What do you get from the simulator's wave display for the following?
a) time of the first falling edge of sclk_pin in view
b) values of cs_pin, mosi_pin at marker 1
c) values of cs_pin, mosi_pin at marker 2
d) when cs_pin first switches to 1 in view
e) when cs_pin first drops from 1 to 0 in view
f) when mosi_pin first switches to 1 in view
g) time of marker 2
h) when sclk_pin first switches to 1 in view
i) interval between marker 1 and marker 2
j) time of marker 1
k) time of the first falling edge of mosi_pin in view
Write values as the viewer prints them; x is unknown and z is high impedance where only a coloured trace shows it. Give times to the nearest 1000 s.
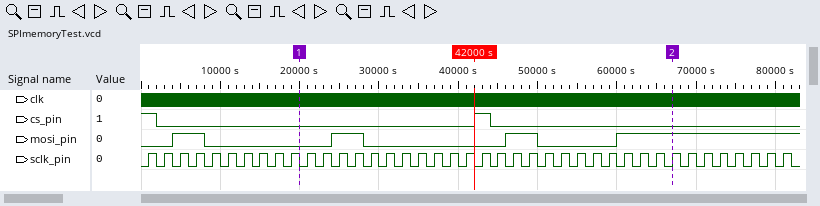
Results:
2000 s
cs_pin=0, mosi_pin=0
cs_pin=0, mosi_pin=1
42000 s
2000 s
4000 s
67000 s
1000 s
47000 s
20000 s
8000 s
